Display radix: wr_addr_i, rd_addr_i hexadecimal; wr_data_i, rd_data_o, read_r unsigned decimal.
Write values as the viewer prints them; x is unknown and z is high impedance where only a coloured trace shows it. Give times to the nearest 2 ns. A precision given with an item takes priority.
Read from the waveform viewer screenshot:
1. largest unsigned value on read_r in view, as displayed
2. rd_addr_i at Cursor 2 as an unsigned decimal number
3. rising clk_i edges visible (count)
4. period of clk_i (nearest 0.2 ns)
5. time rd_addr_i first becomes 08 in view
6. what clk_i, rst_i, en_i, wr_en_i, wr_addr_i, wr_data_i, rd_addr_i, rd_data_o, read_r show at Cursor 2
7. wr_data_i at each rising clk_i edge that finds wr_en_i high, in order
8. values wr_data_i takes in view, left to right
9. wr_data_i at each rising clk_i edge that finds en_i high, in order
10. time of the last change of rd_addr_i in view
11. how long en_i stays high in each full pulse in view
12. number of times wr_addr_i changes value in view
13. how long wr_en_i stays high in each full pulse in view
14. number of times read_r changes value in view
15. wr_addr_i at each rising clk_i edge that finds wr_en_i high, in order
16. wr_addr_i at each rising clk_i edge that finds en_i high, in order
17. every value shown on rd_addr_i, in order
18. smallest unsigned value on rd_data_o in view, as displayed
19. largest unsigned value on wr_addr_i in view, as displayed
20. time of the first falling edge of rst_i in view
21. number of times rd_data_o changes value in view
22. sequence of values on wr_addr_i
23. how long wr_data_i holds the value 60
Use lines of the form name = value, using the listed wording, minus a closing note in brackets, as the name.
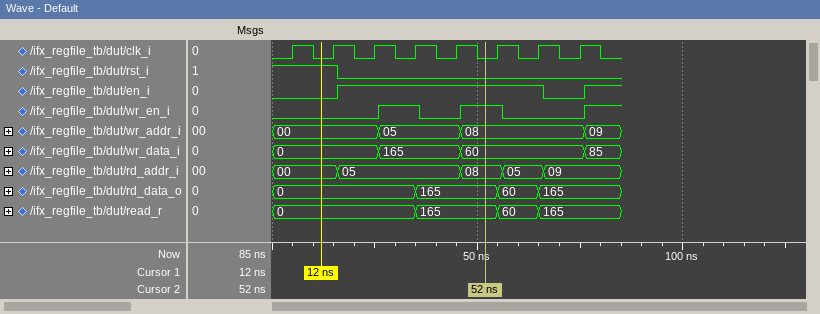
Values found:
largest unsigned value on read_r in view, as displayed = 165
rd_addr_i at Cursor 2 as an unsigned decimal number = 8
rising clk_i edges visible = 8
period of clk_i = 10 ns
time rd_addr_i first becomes 08 in view = 46 ns
what clk_i, rst_i, en_i, wr_en_i, wr_addr_i, wr_data_i, rd_addr_i, rd_data_o, read_r show at Cursor 2 = clk_i=0, rst_i=0, en_i=1, wr_en_i=1, wr_addr_i=08, wr_data_i=60, rd_addr_i=08, rd_data_o=165, read_r=165
wr_data_i at each rising clk_i edge that finds wr_en_i high, in order = 165, 60
values wr_data_i takes in view, left to right = 0, 165, 60, 85
wr_data_i at each rising clk_i edge that finds en_i high, in order = 0, 165, 165, 60, 60
time of the last change of rd_addr_i in view = 66 ns
how long en_i stays high in each full pulse in view = 50 ns
number of times wr_addr_i changes value in view = 3
how long wr_en_i stays high in each full pulse in view = 10 ns, 10 ns
number of times read_r changes value in view = 3
wr_addr_i at each rising clk_i edge that finds wr_en_i high, in order = 05, 08
wr_addr_i at each rising clk_i edge that finds en_i high, in order = 00, 05, 05, 08, 08
every value shown on rd_addr_i, in order = 00, 05, 08, 05, 09
smallest unsigned value on rd_data_o in view, as displayed = 0
largest unsigned value on wr_addr_i in view, as displayed = 09
time of the first falling edge of rst_i in view = 16 ns
number of times rd_data_o changes value in view = 3
sequence of values on wr_addr_i = 00, 05, 08, 09
how long wr_data_i holds the value 60 = 30 ns
